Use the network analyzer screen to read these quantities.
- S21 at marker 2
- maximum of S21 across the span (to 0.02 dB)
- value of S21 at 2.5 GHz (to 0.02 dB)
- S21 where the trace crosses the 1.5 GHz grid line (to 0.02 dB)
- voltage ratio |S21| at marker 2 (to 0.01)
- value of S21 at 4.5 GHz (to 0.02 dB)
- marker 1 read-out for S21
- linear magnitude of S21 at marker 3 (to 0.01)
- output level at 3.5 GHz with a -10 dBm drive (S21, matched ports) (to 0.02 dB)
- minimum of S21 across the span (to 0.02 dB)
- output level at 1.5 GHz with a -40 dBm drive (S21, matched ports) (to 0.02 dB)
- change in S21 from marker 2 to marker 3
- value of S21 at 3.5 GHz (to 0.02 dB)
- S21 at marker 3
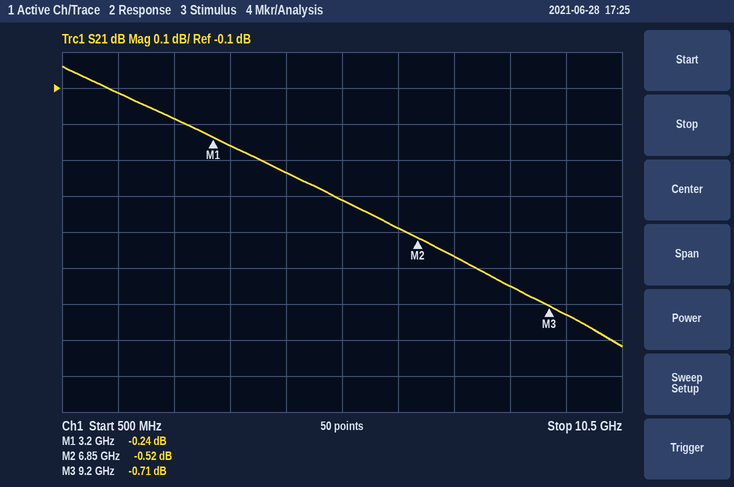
-0.52 dB
-0.04 dB
-0.18 dB
-0.12 dB
0.94
-0.34 dB
-0.24 dB
0.92
-10.26 dBm
-0.82 dB
-40.12 dBm
-0.19 dB
-0.26 dB
-0.71 dB
